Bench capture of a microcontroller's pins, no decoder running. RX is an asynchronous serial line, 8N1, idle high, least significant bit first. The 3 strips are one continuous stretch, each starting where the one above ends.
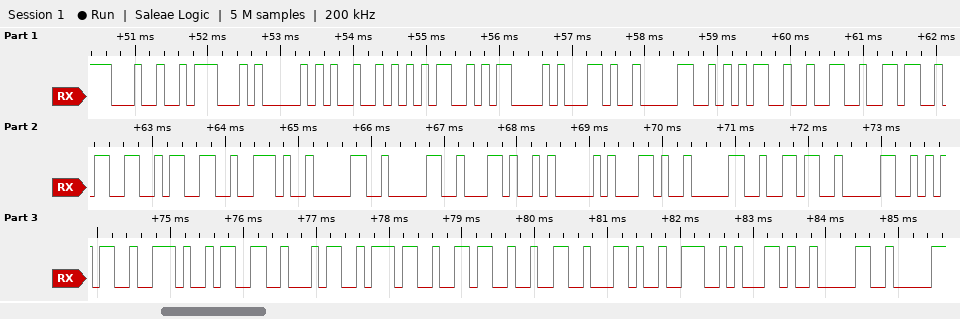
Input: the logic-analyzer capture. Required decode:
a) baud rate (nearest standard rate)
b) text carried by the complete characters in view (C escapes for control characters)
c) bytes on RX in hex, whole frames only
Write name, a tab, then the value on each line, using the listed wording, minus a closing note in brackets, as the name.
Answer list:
baud rate	9600 baud
text carried by the complete characters in view	"$GPRMC,052633.00,A,0605.34762,N,0"
bytes on RX in hex, whole frames only	24 47 50 52 4D 43 2C 30 35 32 36 33 33 2E 30 30 2C 41 2C 30 36 30 35 2E 33 34 37 36 32 2C 4E 2C 30
